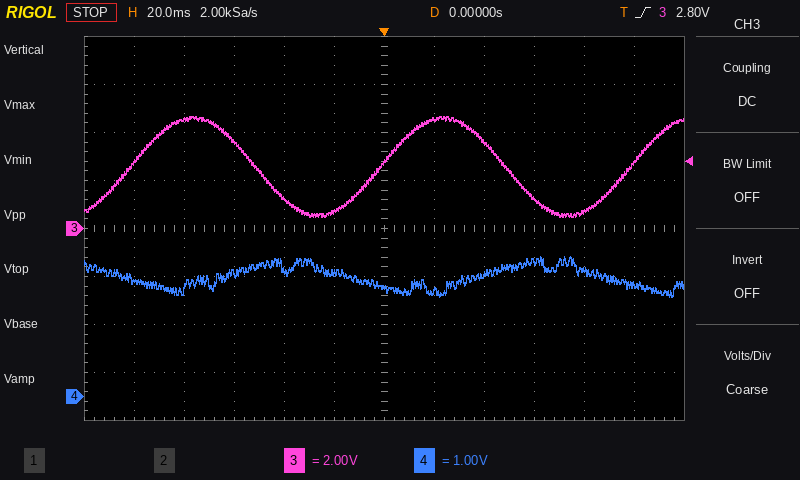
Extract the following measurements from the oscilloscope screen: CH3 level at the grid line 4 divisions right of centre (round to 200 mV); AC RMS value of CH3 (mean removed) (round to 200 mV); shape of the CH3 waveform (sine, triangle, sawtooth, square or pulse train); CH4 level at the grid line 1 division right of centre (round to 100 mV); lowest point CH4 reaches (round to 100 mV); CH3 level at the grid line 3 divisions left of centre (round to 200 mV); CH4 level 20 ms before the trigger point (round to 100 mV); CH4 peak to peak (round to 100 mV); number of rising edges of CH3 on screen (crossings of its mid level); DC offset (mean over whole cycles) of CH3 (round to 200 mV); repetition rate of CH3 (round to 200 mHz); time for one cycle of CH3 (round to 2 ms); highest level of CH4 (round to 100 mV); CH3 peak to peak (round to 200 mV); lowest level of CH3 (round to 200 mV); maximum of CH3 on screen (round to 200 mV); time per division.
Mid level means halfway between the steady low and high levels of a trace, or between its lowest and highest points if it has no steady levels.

800 mV
1.4 V
sine
2.2 V
2.1 V
3.6 V
2.6 V
800 mV
3
2.6 V
10.0 Hz
100 ms
2.9 V
4.2 V
400 mV
4.6 V
20 ms
